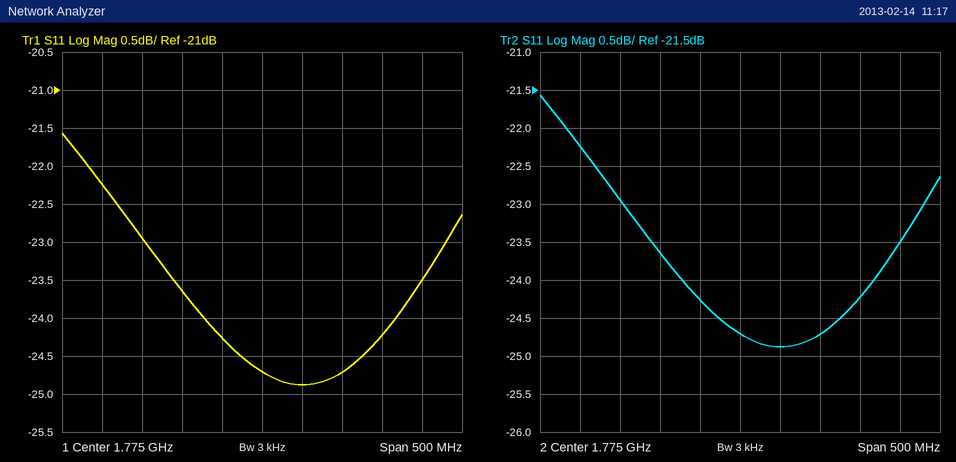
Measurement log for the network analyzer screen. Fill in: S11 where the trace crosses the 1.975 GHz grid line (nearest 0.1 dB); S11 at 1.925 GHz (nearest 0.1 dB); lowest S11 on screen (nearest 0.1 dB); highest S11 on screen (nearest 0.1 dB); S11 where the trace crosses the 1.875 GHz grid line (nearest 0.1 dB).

-23.5 dB
-24.2 dB
-24.9 dB
-21.6 dB
-24.7 dB
